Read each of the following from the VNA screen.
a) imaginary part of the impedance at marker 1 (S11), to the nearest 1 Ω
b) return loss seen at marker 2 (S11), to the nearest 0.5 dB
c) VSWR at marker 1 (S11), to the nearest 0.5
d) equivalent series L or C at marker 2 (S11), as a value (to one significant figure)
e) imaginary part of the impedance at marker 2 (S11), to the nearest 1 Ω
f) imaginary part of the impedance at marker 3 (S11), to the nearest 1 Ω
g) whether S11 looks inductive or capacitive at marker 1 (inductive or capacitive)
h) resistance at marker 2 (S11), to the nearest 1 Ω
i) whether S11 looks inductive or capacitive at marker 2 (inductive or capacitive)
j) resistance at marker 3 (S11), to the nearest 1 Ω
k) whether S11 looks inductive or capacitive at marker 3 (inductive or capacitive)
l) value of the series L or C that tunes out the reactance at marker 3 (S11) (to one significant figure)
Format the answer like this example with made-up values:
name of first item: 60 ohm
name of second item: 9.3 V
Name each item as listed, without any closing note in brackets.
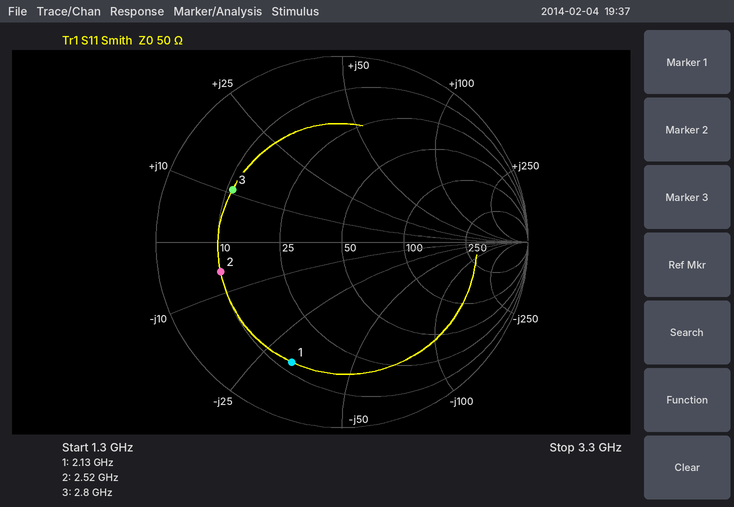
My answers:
imaginary part of the impedance at marker 1 (S11), to the nearest 1 Ω: -32 Ω
return loss seen at marker 2 (S11), to the nearest 0.5 dB: 3.5 dB
VSWR at marker 1 (S11), to the nearest 0.5: 5.5
equivalent series L or C at marker 2 (S11), as a value: 10 pF
imaginary part of the impedance at marker 2 (S11), to the nearest 1 Ω: -6 Ω
imaginary part of the impedance at marker 3 (S11), to the nearest 1 Ω: +11 Ω
whether S11 looks inductive or capacitive at marker 1: capacitive
resistance at marker 2 (S11), to the nearest 1 Ω: 10 Ω
whether S11 looks inductive or capacitive at marker 2: capacitive
resistance at marker 3 (S11), to the nearest 1 Ω: 11 Ω
whether S11 looks inductive or capacitive at marker 3: inductive
value of the series L or C that tunes out the reactance at marker 3 (S11): 5 pF
